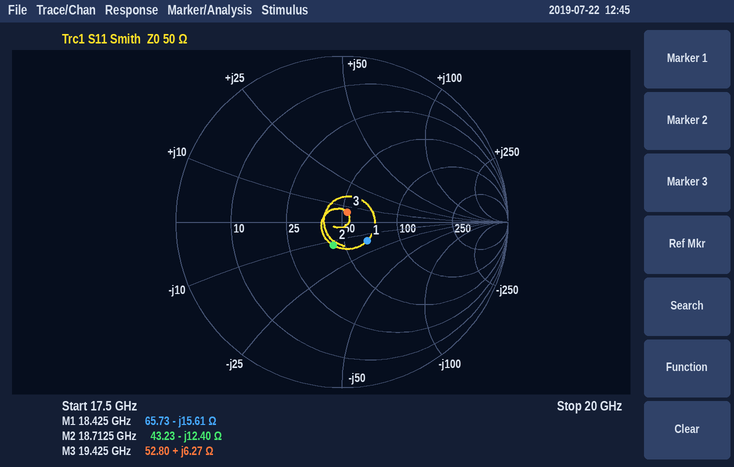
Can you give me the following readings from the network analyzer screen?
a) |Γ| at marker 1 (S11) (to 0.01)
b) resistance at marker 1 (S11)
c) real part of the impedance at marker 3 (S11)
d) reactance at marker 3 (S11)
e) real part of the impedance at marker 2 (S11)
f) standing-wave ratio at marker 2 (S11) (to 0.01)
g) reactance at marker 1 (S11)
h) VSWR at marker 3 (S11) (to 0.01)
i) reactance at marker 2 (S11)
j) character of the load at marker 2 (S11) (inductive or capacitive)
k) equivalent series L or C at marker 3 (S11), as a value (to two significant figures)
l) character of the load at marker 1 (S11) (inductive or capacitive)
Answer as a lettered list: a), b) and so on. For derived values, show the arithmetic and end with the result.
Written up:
a) 0.19
b) 65.73 Ω
c) 52.80 Ω
d) +6.27 Ω
e) 43.23 Ω
f) 1.35
g) -15.61 Ω
h) 1.14
i) -12.40 Ω
j) capacitive
k) L = 6.27 Ω/(2π × 19.425 GHz) ≈ 51 pH
l) capacitive
